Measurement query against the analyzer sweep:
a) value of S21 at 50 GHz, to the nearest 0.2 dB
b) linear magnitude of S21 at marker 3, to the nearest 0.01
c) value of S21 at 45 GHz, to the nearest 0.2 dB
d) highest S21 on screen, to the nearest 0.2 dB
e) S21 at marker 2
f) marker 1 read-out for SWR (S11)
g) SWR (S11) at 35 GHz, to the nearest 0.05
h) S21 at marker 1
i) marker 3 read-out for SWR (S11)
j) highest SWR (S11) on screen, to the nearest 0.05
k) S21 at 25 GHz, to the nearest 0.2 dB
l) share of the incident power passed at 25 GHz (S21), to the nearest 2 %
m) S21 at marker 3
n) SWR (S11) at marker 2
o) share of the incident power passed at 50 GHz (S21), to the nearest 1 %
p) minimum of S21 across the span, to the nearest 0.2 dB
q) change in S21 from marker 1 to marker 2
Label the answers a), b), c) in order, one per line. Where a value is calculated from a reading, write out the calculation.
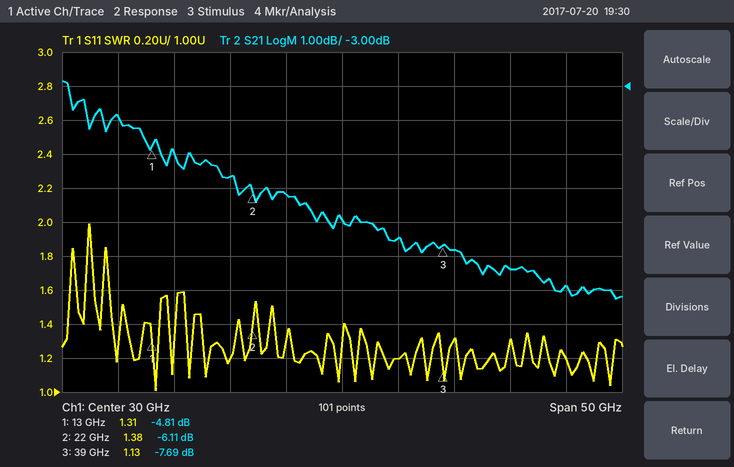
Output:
a) -8.8 dB
b) 10^(-7.69/20) ≈ 0.41
c) -8.4 dB
d) -2.8 dB
e) -6.11 dB
f) 1.31
g) 1.20
h) -4.81 dB
i) 1.13
j) 2.00
k) -6.2 dB
l) 10^(-6.2/10) ≈ 24 %
m) -7.69 dB
n) 1.38
o) 10^(-8.8/10) ≈ 13 %
p) -9.2 dB
q) -6.11 − (-4.81) = -1.30 dB
